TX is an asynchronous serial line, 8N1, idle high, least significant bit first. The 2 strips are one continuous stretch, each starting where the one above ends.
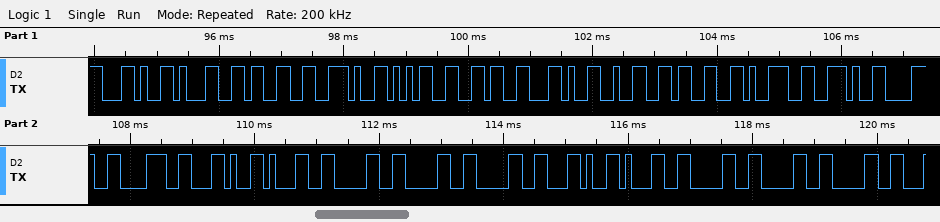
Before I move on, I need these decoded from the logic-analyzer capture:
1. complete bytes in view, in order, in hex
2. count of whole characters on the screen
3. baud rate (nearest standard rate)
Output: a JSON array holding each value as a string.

["2C 31 33 2E 35 36 2C 32 33 39 2E 38 38 2C 31 30 30 30 2C 31 30 30 30", "23", "9600 baud"]
